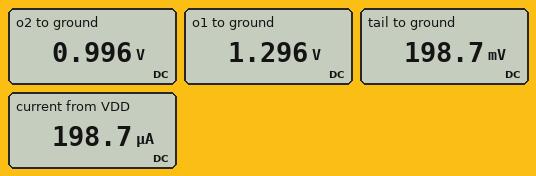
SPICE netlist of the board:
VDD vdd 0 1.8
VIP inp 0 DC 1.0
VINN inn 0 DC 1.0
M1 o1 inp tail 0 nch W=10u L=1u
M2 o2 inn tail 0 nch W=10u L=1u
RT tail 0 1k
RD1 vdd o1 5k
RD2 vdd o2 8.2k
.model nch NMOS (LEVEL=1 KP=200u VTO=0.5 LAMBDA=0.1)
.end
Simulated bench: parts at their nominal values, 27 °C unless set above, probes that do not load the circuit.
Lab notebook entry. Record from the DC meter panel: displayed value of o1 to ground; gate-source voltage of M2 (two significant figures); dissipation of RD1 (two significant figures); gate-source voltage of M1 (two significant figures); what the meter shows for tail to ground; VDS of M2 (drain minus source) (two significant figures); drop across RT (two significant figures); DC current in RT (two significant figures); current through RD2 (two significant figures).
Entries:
1.296 V
800 mV
51 µW
800 mV
198.7 mV
800 mV
200 mV
200 µA
98 µA
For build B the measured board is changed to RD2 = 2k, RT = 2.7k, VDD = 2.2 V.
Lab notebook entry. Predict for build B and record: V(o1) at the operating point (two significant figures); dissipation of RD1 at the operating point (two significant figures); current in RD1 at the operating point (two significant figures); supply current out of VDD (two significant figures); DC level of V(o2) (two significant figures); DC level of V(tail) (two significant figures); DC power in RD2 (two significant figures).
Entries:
1.9 V
14 µW
53 µA
110 µA
2.1 V
290 mV
5.7 µW
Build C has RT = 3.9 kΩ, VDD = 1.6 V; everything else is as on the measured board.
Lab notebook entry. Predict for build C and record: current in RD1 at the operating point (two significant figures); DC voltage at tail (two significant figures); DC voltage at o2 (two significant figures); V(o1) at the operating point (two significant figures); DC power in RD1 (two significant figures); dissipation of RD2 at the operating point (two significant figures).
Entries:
40 µA
310 mV
1.3 V
1.4 V
8.0 µW
13 µW
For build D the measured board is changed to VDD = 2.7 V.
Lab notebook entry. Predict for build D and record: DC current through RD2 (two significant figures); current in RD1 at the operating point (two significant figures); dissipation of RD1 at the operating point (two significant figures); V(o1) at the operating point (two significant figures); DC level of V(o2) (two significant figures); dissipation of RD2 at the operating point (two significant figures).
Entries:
100 µA
100 µA
54 µW
2.2 V
1.9 V
84 µW
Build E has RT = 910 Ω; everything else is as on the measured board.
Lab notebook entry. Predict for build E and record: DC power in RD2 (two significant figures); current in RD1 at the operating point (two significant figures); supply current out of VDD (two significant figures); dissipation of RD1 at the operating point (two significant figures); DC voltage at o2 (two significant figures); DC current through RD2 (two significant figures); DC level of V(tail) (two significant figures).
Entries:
87 µW
110 µA
210 µA
56 µW
950 mV
100 µA
190 mV
